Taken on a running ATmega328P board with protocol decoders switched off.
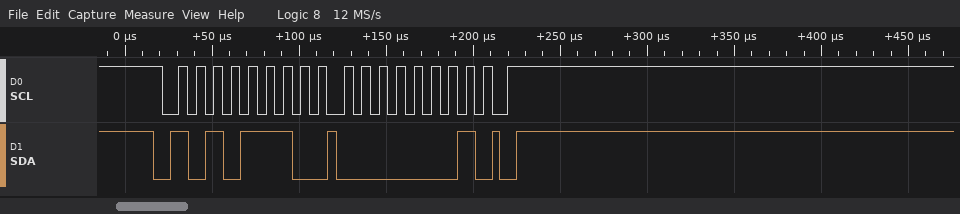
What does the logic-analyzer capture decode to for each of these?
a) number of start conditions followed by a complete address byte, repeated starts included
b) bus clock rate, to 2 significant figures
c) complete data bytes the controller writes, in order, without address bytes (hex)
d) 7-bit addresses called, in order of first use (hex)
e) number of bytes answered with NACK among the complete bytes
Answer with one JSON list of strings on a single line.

["1", "100 kHz", "01", "0x57", "0"]
